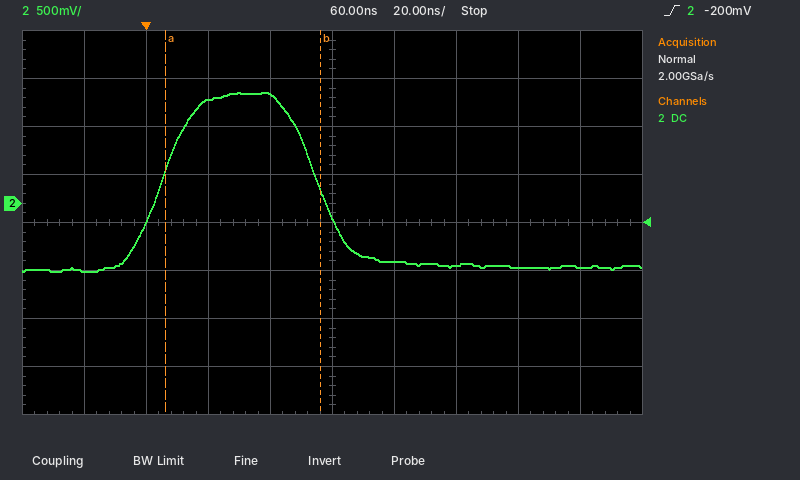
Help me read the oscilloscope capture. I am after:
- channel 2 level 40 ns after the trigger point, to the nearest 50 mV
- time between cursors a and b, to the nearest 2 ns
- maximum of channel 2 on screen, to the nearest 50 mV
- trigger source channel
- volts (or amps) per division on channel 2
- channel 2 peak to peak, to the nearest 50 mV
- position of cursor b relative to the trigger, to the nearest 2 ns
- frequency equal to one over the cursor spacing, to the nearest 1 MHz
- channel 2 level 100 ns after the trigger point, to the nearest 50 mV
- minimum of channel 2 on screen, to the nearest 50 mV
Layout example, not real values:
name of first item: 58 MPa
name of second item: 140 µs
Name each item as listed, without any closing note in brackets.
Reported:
channel 2 level 40 ns after the trigger point, to the nearest 50 mV: 1.15 V
time between cursors a and b, to the nearest 2 ns: 50 ns
maximum of channel 2 on screen, to the nearest 50 mV: 1.15 V
trigger source channel: channel 2
volts (or amps) per division on channel 2: 500 mV
channel 2 peak to peak, to the nearest 50 mV: 1.85 V
position of cursor b relative to the trigger, to the nearest 2 ns: +56 ns
frequency equal to one over the cursor spacing, to the nearest 1 MHz: 20 MHz
channel 2 level 100 ns after the trigger point, to the nearest 50 mV: -650 mV
minimum of channel 2 on screen, to the nearest 50 mV: -700 mV
